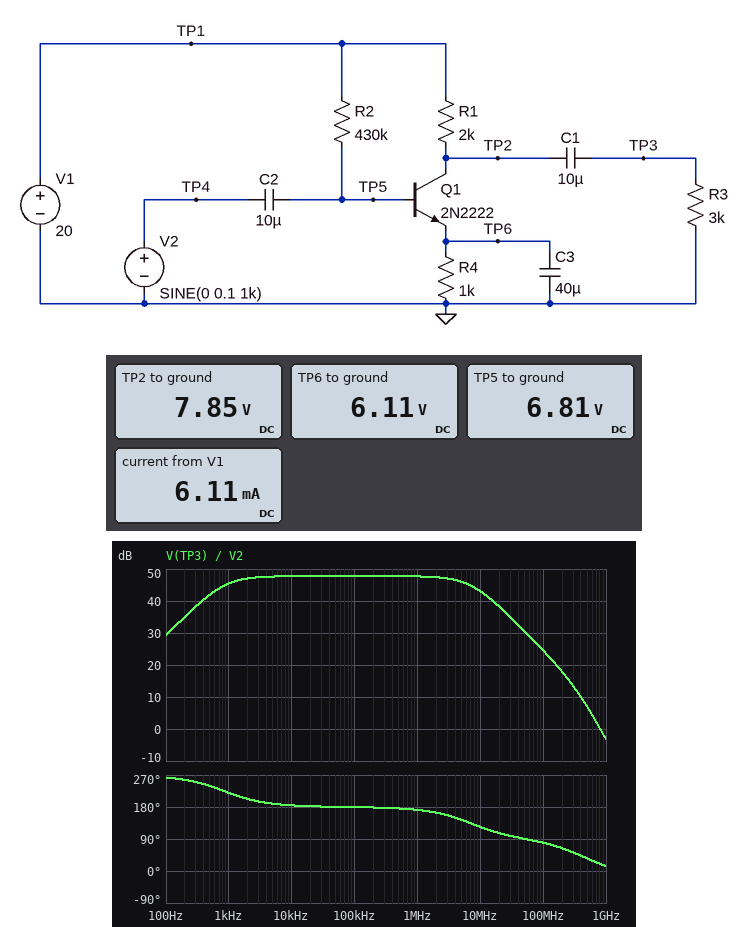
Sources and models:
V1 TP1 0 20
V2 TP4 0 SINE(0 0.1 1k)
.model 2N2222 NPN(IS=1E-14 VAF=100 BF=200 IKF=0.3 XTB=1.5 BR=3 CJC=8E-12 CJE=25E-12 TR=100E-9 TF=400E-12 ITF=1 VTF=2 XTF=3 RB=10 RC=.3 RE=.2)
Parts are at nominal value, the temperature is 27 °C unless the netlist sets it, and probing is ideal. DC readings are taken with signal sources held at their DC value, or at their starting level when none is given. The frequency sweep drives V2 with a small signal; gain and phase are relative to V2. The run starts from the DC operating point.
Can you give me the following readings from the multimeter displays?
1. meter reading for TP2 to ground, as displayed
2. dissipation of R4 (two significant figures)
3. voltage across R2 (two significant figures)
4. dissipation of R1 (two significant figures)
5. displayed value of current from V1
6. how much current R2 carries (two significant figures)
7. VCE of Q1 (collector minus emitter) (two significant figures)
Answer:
7.85 V
37 mW
13 V
74 mW
6.11 mA
31 µA
1.7 V
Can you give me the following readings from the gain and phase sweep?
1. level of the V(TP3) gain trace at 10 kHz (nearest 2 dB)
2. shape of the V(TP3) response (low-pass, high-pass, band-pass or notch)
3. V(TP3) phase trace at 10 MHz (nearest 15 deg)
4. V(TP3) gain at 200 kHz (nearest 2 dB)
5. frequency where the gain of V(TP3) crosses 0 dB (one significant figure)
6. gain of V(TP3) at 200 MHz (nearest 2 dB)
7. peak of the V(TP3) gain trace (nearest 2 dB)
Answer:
48 dB
band-pass
120 deg
48 dB
800 MHz
18 dB
48 dB
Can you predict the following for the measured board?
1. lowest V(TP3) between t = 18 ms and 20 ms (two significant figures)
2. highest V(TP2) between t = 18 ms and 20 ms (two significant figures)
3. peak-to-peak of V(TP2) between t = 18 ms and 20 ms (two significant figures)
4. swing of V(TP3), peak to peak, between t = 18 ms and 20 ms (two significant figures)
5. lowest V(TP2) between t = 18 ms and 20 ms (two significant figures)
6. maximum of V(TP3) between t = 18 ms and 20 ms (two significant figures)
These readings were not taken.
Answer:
-4.1 V
16 V
10 V
10 V
5.3 V
6.3 V
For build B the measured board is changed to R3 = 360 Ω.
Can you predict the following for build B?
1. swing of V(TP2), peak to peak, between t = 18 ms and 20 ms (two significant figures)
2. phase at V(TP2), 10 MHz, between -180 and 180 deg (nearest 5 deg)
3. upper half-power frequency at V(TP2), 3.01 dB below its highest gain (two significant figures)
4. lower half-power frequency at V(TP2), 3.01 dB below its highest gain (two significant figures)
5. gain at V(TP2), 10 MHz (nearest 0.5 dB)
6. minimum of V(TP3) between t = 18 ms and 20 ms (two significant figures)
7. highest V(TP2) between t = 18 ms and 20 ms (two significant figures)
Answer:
4.8 V
155 deg
24 MHz
880 Hz
35.5 dB
-3.2 V
11 V
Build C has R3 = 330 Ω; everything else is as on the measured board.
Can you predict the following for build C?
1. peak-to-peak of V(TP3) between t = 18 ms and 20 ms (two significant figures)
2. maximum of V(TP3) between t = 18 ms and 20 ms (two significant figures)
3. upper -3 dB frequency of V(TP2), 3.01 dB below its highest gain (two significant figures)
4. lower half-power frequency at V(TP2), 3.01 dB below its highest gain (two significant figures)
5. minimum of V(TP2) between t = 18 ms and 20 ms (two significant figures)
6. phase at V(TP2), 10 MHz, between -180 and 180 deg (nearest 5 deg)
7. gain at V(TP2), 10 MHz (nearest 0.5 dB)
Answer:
4.6 V
1.6 V
25 MHz
880 Hz
5.9 V
155 deg
35.0 dB
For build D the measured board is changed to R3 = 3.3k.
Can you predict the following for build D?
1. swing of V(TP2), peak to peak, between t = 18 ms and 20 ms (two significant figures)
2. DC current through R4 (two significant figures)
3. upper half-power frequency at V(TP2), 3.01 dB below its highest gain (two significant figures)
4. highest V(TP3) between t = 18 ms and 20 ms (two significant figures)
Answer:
11 V
6.1 mA
6.9 MHz
6.6 V
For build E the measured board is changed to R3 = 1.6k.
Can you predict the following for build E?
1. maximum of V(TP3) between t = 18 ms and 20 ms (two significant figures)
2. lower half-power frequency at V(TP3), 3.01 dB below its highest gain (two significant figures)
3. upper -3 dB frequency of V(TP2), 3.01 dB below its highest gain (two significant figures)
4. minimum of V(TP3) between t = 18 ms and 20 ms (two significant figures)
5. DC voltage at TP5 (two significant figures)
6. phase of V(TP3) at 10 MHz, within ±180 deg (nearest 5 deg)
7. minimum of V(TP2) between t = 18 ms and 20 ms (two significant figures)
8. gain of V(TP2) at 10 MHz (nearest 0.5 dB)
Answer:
4.6 V
850 Hz
9.3 MHz
-4.3 V
6.8 V
130 deg
5.4 V
42.0 dB
